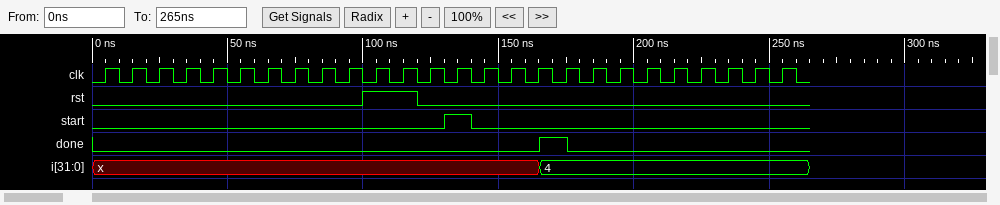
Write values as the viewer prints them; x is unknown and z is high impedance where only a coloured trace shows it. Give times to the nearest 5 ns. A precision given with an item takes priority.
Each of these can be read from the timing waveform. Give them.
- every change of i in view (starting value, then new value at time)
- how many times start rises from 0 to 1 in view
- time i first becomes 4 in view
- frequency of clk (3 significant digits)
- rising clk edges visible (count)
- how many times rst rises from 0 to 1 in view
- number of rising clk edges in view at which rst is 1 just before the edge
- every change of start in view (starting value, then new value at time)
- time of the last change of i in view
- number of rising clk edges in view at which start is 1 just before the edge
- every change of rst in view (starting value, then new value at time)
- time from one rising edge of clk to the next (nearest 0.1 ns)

x, 4 at 165 ns
1
165 ns
100 MHz
26
1
2
0, 1 at 130 ns, 0 at 140 ns
165 ns
1
0, 1 at 100 ns, 0 at 120 ns
10 ns
